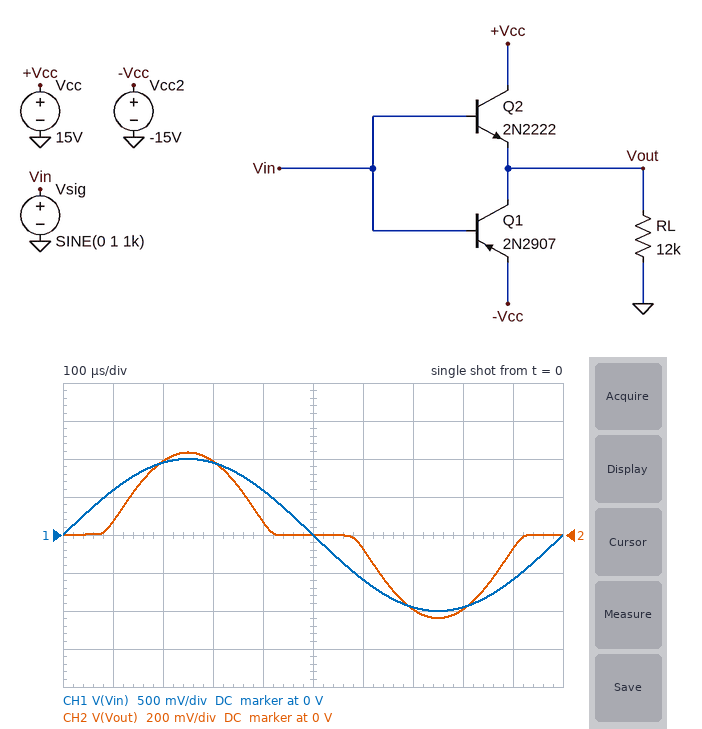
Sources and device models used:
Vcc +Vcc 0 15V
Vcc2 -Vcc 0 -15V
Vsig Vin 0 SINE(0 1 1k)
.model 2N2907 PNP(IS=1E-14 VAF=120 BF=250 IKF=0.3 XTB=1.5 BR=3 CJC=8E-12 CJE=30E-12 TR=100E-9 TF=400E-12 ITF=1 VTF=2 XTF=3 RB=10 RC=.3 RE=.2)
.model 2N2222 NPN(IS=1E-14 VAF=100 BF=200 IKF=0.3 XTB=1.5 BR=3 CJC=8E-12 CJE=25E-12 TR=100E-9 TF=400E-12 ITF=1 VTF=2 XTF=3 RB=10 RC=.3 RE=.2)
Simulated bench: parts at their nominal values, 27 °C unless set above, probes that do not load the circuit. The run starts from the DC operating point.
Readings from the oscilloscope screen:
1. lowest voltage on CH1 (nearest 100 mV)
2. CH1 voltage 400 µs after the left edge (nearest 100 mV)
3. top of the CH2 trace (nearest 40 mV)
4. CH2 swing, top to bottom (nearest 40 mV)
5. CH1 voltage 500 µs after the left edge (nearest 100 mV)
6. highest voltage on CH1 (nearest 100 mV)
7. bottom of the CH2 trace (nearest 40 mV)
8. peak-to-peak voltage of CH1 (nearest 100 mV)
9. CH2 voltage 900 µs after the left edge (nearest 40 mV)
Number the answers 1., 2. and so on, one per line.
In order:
1. -1.0 V
2. 600 mV
3. 440 mV
4. 880 mV
5. 0 V
6. 1.0 V
7. -440 mV
8. 2.0 V
9. -80 mV
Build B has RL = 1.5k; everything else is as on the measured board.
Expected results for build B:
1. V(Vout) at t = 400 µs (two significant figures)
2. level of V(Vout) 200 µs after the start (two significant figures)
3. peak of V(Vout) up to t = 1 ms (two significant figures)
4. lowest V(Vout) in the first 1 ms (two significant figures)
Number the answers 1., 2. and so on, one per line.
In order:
1. 34 mV
2. 340 mV
3. 380 mV
4. -390 mV
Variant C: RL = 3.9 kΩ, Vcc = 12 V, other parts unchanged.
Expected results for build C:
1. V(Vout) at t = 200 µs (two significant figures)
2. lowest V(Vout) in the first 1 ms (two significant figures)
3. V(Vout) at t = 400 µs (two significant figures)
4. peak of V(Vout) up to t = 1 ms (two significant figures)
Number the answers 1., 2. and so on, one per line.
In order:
1. 360 mV
2. -410 mV
3. 49 mV
4. 410 mV
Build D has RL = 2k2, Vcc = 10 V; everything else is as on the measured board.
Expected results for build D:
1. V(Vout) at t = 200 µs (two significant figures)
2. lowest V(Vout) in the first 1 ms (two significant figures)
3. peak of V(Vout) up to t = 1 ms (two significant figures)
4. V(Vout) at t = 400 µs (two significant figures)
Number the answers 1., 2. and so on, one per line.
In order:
1. 350 mV
2. -400 mV
3. 390 mV
4. 39 mV
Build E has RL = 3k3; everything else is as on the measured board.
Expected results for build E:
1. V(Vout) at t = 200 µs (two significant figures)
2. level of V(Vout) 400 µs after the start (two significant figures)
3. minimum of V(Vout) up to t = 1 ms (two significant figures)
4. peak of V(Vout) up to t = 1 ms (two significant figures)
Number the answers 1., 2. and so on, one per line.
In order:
1. 360 mV
2. 46 mV
3. -410 mV
4. 400 mV
